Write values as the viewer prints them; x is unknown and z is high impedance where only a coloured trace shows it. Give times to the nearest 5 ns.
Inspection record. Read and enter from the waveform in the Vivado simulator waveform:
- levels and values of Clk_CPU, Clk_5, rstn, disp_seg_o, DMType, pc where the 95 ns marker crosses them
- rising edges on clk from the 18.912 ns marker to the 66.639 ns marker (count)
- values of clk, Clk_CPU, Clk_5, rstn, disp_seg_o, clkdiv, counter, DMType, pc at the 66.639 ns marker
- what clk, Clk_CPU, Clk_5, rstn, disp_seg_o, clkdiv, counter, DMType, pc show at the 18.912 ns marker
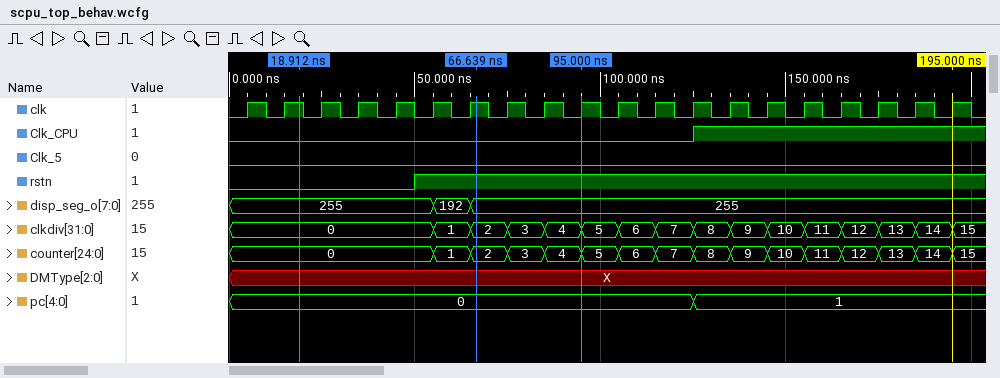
Clk_CPU=0, Clk_5=0, rstn=1, disp_seg_o=255, DMType=X, pc=0
5
clk=1, Clk_CPU=0, Clk_5=0, rstn=1, disp_seg_o=255, clkdiv=2, counter=2, DMType=X, pc=0
clk=1, Clk_CPU=0, Clk_5=0, rstn=0, disp_seg_o=255, clkdiv=0, counter=0, DMType=X, pc=0
